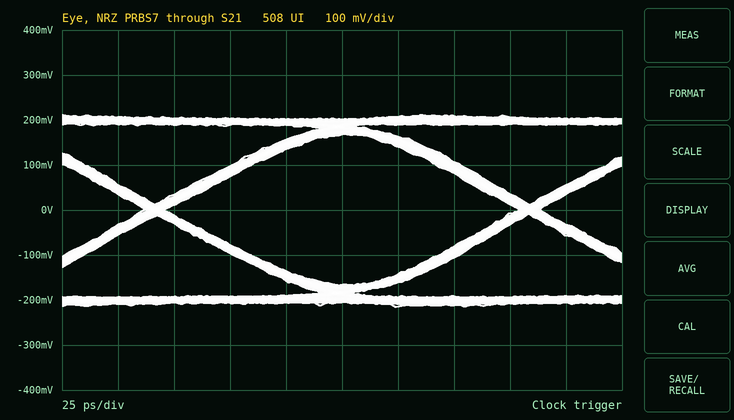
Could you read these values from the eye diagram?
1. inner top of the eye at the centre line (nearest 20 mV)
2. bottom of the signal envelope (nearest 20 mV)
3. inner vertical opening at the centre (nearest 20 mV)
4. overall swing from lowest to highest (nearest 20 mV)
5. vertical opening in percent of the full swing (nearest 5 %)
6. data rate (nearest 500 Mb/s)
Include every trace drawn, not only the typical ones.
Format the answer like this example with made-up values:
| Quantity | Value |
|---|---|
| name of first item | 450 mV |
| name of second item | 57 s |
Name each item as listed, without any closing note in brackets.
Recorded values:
| Quantity | Value |
|---|---|
| inner top of the eye at the centre line | 160 mV |
| bottom of the signal envelope | -220 mV |
| inner vertical opening at the centre | 340 mV |
| overall swing from lowest to highest | 420 mV |
| vertical opening in percent of the full swing | 80 % |
| data rate | 6.0 Gb/s |
